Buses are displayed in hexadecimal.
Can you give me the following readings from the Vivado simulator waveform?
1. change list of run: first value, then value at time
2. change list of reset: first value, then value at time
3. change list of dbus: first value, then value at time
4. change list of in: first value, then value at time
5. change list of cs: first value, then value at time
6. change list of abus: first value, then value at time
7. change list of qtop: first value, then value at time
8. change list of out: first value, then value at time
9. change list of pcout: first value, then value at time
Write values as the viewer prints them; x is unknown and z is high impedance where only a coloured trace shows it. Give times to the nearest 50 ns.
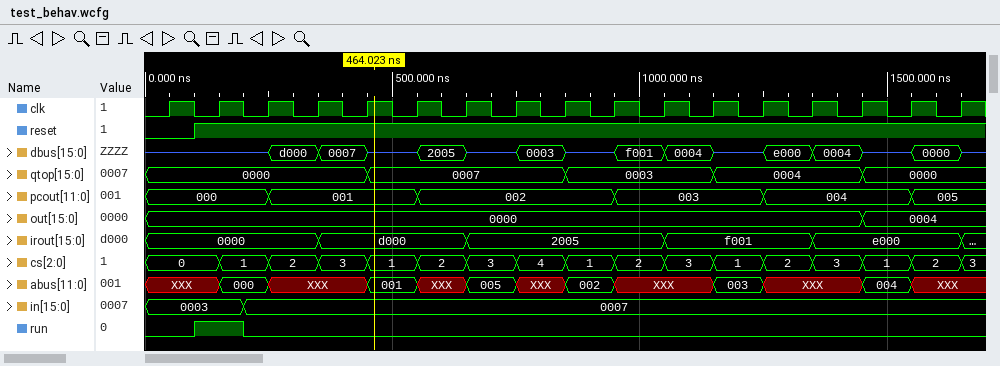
0, 1 at 100 ns, 0 at 200 ns
0, 1 at 100 ns
z, d000 at 250 ns, 0007 at 350 ns, z at 450 ns, 2005 at 550 ns, z at 650 ns, 0003 at 750 ns, z at 850 ns, f001 at 950 ns, 0004 at 1050 ns, z at 1150 ns, e000 at 1250 ns, 0004 at 1350 ns, z at 1450 ns, 0000 at 1550 ns, z at 1650 ns
0003, 0007 at 200 ns
0, 1 at 150 ns, 2 at 250 ns, 3 at 350 ns, 1 at 450 ns, 2 at 550 ns, 3 at 650 ns, 4 at 750 ns, 1 at 850 ns, 2 at 950 ns, 3 at 1050 ns, 1 at 1150 ns, 2 at 1250 ns, 3 at 1350 ns, 1 at 1450 ns, 2 at 1550 ns, 3 at 1650 ns
XXX, 000 at 150 ns, XXX at 250 ns, 001 at 450 ns, XXX at 550 ns, 005 at 650 ns, XXX at 750 ns, 002 at 850 ns, XXX at 950 ns, 003 at 1150 ns, XXX at 1250 ns, 004 at 1450 ns, XXX at 1550 ns
0000, 0007 at 450 ns, 0003 at 850 ns, 0004 at 1150 ns, 0000 at 1450 ns
0000, 0004 at 1450 ns
000, 001 at 250 ns, 002 at 550 ns, 003 at 950 ns, 004 at 1250 ns, 005 at 1550 ns
